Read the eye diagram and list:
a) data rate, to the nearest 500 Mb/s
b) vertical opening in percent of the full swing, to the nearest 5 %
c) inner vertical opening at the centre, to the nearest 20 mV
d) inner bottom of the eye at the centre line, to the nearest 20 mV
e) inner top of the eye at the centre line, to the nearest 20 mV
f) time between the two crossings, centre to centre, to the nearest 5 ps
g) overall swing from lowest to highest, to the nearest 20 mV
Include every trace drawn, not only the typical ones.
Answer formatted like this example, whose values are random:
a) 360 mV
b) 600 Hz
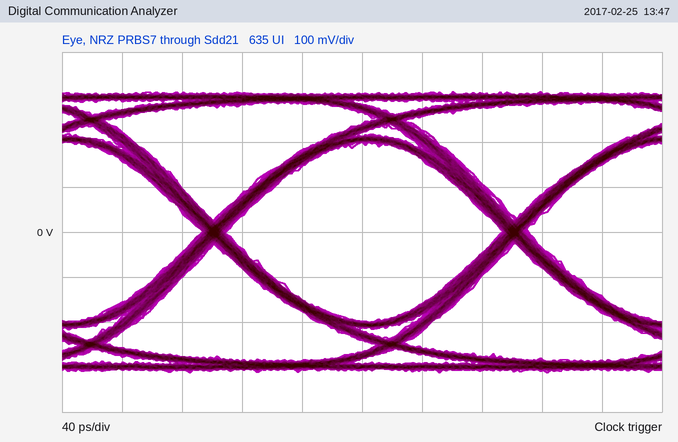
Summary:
a) 5.0 Gb/s
b) 65 %
c) 400 mV
d) -200 mV
e) 200 mV
f) 200 ps
g) 620 mV
